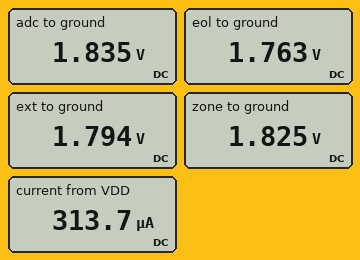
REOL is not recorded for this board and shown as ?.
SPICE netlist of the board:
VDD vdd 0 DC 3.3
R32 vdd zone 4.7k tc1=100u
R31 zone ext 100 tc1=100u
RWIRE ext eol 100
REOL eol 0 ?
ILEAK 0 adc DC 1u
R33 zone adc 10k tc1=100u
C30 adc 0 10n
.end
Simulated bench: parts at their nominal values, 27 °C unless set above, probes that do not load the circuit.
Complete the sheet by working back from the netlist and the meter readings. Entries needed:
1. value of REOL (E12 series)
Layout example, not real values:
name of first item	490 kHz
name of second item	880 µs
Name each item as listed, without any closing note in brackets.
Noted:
value of REOL	5.6 kΩ
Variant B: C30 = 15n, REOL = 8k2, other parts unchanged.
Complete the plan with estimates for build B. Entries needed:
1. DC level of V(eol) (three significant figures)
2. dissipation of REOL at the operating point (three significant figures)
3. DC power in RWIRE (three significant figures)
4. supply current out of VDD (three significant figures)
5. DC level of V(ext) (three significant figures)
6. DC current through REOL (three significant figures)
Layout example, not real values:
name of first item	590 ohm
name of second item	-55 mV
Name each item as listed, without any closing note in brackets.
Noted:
DC level of V(eol)	2.07 V
dissipation of REOL at the operating point	522 µW
DC power in RWIRE	6.36 µW
supply current out of VDD	251 µA
DC level of V(ext)	2.09 V
DC current through REOL	252 µA
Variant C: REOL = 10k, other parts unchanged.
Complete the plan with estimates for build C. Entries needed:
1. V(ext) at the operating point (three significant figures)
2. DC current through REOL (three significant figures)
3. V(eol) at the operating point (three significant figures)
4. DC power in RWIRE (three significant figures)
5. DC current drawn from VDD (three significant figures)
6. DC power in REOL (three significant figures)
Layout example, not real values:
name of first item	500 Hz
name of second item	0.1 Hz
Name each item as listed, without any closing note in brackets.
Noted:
V(ext) at the operating point	2.24 V
DC current through REOL	222 µA
V(eol) at the operating point	2.22 V
DC power in RWIRE	4.92 µW
DC current drawn from VDD	221 µA
DC power in REOL	492 µW
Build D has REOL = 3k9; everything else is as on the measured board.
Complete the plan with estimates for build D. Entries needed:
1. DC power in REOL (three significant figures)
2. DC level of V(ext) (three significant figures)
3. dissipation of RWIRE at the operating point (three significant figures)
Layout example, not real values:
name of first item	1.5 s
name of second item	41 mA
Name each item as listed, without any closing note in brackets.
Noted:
DC power in REOL	550 µW
DC level of V(ext)	1.50 V
dissipation of RWIRE at the operating point	14.1 µW
